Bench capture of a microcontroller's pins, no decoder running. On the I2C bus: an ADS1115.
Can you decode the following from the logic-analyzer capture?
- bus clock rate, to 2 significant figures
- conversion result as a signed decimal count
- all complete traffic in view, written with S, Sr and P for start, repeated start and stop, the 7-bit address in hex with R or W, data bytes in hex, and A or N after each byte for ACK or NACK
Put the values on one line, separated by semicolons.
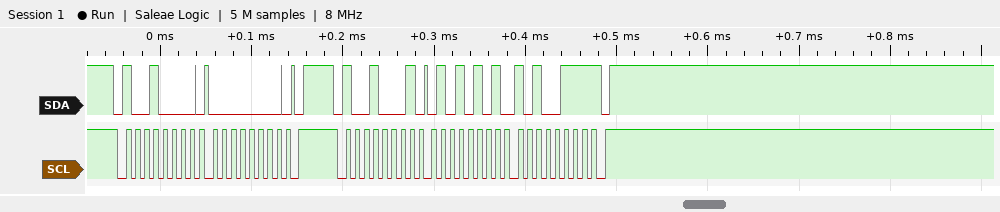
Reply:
100 kHz; 21927; S 48W A 00 A P S 48R A 55 A A7 N P
